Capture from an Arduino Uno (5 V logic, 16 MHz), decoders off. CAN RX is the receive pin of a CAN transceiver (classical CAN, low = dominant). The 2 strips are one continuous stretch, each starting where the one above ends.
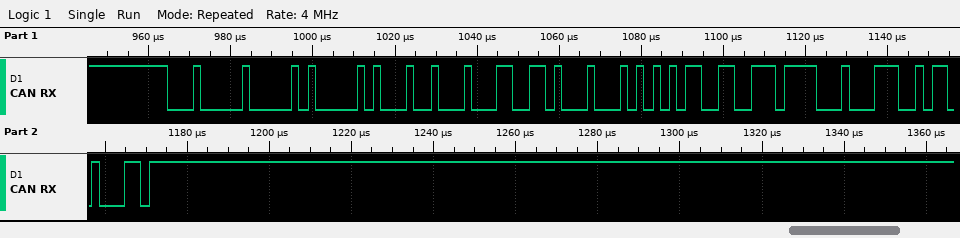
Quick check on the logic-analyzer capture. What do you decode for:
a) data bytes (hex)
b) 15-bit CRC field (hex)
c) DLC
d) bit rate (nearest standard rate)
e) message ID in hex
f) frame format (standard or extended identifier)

11 22 33 44 55 66 77 88
0x72D1
8
500 kbit/s
0x100
standard
